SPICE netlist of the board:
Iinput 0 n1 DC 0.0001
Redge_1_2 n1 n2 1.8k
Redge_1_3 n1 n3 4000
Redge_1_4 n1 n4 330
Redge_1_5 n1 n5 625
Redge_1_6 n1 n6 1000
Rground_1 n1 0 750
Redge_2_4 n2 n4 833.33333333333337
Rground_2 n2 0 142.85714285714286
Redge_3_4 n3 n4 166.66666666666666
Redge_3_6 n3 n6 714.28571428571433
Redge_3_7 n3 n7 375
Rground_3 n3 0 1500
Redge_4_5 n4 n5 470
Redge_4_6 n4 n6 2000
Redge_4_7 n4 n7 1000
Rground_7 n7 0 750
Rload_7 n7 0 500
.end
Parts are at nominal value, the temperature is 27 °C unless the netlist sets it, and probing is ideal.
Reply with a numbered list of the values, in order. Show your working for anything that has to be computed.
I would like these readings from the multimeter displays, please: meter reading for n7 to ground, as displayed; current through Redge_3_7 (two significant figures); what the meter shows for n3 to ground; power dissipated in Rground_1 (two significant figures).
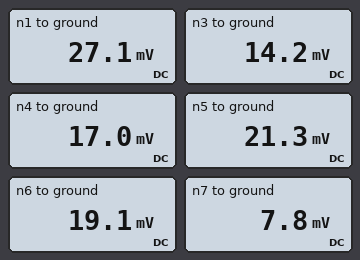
1. 7.8 mV
2. (14.2 mV - 7.8 mV) / 375 Ω = 17 µA
3. 14.2 mV
4. (27.1 mV)^2 / 750 Ω = 980 nW
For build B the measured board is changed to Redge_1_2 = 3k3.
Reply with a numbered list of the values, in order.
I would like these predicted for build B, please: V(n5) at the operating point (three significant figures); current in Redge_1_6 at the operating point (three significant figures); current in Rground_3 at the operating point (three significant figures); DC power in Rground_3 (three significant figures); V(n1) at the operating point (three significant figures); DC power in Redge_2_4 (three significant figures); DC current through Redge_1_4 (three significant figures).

1. 22.4 mV
2. 8.44 µA
3. 9.93 µA
4. 148 nW
5. 28.5 mV
6. 243 nW
7. 32.7 µA
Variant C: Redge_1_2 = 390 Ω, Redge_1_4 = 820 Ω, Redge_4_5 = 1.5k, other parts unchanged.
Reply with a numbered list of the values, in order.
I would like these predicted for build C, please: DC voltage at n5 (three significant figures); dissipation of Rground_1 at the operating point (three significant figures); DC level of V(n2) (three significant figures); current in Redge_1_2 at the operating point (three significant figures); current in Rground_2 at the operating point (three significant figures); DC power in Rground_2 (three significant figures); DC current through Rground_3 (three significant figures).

1. 19.1 mV
2. 664 nW
3. 6.57 mV
4. 40.4 µA
5. 46.0 µA
6. 302 nW
7. 6.51 µA
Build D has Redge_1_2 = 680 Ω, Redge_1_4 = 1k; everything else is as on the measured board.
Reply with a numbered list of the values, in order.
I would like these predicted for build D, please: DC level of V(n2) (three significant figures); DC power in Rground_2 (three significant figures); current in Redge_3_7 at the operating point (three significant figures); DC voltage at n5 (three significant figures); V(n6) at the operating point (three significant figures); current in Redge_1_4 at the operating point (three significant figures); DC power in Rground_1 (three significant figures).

1. 5.47 mV
2. 209 nW
3. 13.6 µA
4. 18.3 mV
5. 16.4 mV
6. 12.6 µA
7. 864 nW
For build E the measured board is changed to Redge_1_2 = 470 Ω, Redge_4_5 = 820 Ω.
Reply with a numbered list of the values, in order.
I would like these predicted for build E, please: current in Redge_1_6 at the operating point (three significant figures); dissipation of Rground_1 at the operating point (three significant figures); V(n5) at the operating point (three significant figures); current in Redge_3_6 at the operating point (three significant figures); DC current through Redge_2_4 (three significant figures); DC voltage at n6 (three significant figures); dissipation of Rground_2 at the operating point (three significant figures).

1. 6.24 µA
2. 623 nW
3. 18.2 mV
4. 5.42 µA
5. 9.24 µA
6. 15.4 mV
7. 256 nW
